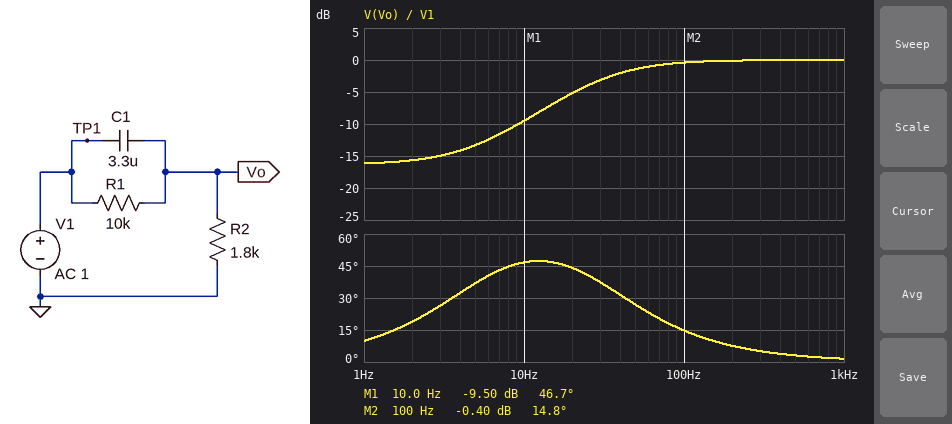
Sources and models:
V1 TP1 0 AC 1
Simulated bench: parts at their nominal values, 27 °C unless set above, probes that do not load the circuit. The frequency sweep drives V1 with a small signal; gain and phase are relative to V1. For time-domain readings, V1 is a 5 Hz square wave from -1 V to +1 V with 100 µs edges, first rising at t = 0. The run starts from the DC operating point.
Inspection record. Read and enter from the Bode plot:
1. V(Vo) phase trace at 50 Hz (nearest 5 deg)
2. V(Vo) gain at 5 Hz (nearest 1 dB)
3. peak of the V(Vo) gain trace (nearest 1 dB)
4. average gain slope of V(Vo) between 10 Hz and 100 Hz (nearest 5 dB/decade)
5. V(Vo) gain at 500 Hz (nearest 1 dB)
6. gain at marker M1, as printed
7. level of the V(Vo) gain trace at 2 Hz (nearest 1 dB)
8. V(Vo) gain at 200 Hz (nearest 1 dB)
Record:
25 deg
-13 dB
0 dB
10 dB/decade
0 dB
-9.50 dB
-16 dB
0 dB
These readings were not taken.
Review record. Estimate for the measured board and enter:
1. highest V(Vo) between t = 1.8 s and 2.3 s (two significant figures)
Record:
1.8 V
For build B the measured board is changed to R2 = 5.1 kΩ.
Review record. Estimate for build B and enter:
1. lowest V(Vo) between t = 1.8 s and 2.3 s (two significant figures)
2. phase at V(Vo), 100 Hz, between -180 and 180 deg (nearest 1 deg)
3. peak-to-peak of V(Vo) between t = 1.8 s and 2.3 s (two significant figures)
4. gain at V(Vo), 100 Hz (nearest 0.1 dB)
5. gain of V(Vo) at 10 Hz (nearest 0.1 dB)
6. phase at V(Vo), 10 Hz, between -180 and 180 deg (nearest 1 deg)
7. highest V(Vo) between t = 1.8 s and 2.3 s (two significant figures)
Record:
-1.7 V
5 deg
3.3 V
-0.1 dB
-3.9 dB
29 deg
1.7 V
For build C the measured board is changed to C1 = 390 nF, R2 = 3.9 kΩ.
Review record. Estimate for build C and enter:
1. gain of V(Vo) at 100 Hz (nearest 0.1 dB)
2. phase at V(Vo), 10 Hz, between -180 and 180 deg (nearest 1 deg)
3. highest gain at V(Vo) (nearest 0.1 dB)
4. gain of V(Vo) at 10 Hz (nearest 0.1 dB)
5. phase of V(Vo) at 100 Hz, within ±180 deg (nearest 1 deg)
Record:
-4.3 dB
10 deg
0 dB
-10.8 dB
33 deg
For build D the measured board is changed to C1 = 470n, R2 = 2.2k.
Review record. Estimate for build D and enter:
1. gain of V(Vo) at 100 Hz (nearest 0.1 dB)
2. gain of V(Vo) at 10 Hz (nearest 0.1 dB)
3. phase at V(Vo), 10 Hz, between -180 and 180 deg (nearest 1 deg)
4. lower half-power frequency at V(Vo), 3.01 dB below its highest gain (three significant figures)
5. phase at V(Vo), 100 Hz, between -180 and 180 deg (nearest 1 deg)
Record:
-6.1 dB
-14.5 dB
13 deg
182 Hz
43 deg
